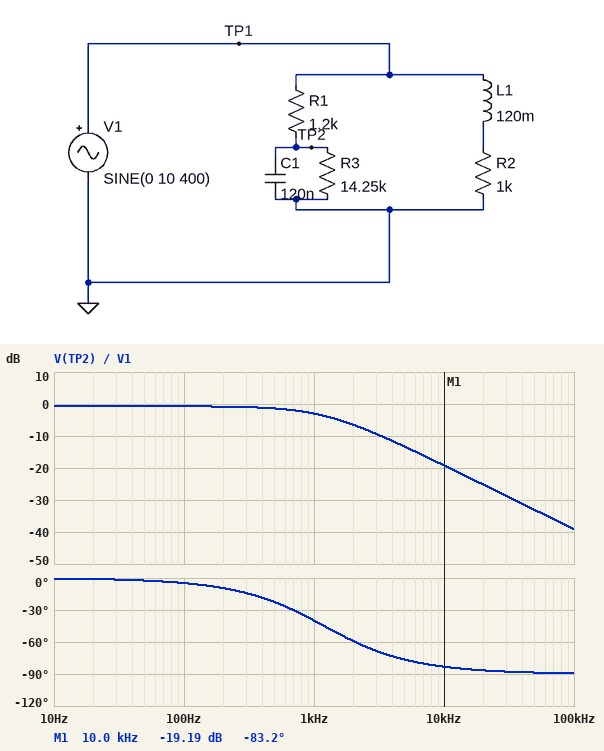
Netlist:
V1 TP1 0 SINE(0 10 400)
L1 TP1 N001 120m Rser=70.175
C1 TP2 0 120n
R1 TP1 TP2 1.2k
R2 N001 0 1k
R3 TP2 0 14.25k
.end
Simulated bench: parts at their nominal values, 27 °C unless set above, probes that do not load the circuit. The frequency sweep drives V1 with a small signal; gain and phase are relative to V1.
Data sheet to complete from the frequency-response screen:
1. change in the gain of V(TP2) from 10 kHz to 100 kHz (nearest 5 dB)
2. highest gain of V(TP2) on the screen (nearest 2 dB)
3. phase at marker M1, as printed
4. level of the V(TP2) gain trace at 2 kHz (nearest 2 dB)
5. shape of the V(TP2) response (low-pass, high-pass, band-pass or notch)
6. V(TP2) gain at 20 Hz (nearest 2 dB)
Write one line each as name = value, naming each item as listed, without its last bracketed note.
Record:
change in the gain of V(TP2) from 10 kHz to 100 kHz = -20 dB
highest gain of V(TP2) on the screen = 0 dB
phase at marker M1, as printed = -83.2 deg
level of the V(TP2) gain trace at 2 kHz = -6 dB
shape of the V(TP2) response = low-pass
V(TP2) gain at 20 Hz = 0 dB
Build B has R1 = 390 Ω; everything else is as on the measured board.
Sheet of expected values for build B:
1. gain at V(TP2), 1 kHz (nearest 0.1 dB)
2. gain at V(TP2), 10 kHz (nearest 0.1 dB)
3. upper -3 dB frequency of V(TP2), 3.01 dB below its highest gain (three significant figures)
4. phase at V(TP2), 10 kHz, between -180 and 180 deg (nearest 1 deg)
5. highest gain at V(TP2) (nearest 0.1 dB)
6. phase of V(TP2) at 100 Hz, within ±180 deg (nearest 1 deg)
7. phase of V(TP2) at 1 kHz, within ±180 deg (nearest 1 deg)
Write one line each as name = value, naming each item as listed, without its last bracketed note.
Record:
gain at V(TP2), 1 kHz = -0.6 dB
gain at V(TP2), 10 kHz = -9.9 dB
upper -3 dB frequency of V(TP2), 3.01 dB below its highest gain = 3.49 kHz
phase at V(TP2), 10 kHz, between -180 and 180 deg = -71 deg
highest gain at V(TP2) = -0.2 dB
phase of V(TP2) at 100 Hz, within ±180 deg = -2 deg
phase of V(TP2) at 1 kHz, within ±180 deg = -16 deg
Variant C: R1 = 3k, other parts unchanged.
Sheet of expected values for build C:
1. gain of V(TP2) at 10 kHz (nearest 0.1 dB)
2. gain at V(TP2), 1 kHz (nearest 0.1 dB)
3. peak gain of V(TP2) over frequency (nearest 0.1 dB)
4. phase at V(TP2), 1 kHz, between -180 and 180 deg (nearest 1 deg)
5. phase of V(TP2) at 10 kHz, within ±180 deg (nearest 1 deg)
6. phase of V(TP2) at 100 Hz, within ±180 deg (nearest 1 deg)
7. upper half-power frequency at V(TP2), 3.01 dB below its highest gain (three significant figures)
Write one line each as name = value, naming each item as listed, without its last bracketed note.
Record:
gain of V(TP2) at 10 kHz = -27.1 dB
gain at V(TP2), 1 kHz = -8.2 dB
peak gain of V(TP2) over frequency = -1.7 dB
phase at V(TP2), 1 kHz, between -180 and 180 deg = -62 deg
phase of V(TP2) at 10 kHz, within ±180 deg = -87 deg
phase of V(TP2) at 100 Hz, within ±180 deg = -11 deg
upper half-power frequency at V(TP2), 3.01 dB below its highest gain = 535 Hz
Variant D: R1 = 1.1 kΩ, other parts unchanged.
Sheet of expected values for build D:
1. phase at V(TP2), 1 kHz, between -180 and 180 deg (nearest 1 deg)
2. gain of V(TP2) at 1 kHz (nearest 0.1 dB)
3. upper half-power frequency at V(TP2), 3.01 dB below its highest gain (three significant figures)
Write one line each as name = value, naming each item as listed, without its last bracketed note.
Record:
phase at V(TP2), 1 kHz, between -180 and 180 deg = -38 deg
gain of V(TP2) at 1 kHz = -2.7 dB
upper half-power frequency at V(TP2), 3.01 dB below its highest gain = 1.30 kHz
